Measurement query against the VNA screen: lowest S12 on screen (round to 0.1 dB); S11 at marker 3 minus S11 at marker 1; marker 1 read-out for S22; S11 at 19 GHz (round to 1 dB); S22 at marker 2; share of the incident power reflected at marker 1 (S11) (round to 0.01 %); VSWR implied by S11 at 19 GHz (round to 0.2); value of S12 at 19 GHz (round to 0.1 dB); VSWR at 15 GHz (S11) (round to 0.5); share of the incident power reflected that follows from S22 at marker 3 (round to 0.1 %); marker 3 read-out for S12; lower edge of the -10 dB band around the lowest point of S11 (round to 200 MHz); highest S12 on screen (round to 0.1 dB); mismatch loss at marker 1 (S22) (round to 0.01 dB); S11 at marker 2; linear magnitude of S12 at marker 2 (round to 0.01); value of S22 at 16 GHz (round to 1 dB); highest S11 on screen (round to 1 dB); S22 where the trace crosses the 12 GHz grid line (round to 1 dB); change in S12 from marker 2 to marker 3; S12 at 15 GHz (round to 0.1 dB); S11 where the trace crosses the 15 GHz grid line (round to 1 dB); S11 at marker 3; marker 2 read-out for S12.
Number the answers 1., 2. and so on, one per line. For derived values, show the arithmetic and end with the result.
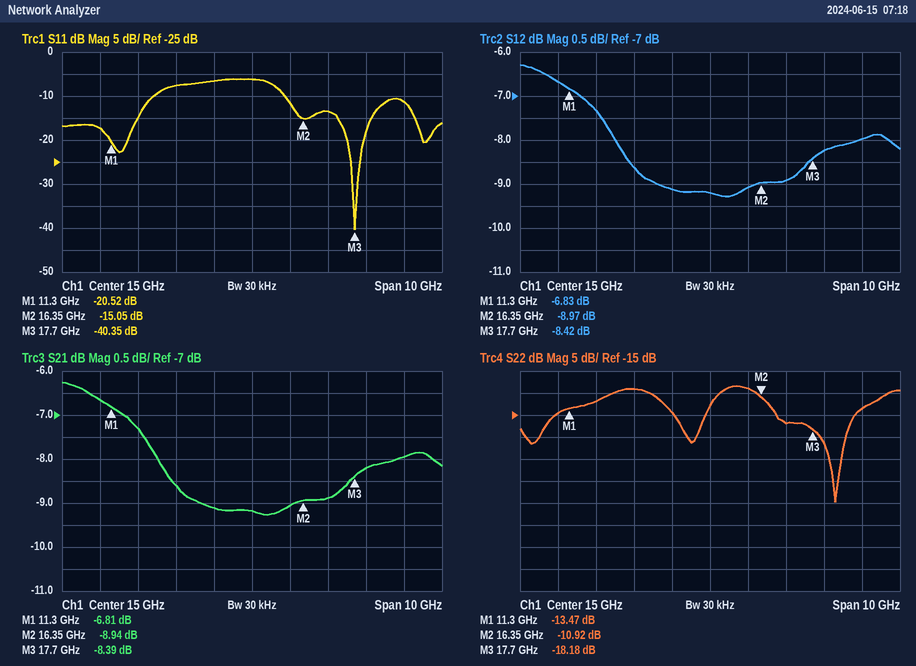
1. -9.3 dB
2. -40.35 − (-20.52) = -19.83 dB
3. -13.47 dB
4. -11 dB
5. -10.92 dB
6. 10^(-20.52/10) ≈ 0.89 %
7. |Γ| = 10^(-11/20) = 0.2818; VSWR = (1 + 0.2818)/(1 − 0.2818) ≈ 1.8
8. -8.0 dB
9. |Γ| = 10^(-6/20) = 0.5012; VSWR = (1 + 0.5012)/(1 − 0.5012) ≈ 3.0
10. 10^(-18.18/10) ≈ 1.5 %
11. -8.42 dB
12. 15.8 GHz
13. -6.3 dB
14. −10 log10(1 − 10^(-13.47/10)) ≈ 0.20 dB
15. -15.05 dB
16. 10^(-8.97/20) ≈ 0.36
17. -9 dB
18. -6 dB
19. -12 dB
20. -8.42 − (-8.97) = 0.55 dB
21. -9.2 dB
22. -6 dB
23. -40.35 dB
24. -8.97 dB
